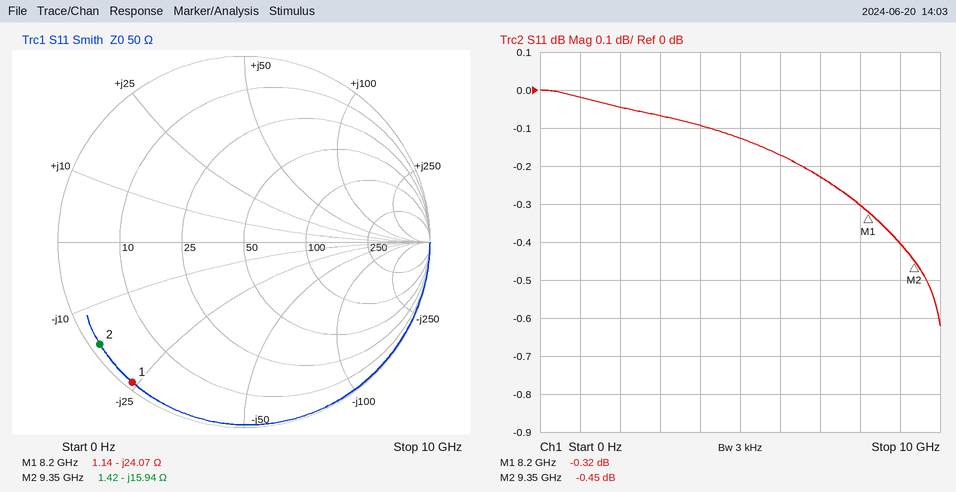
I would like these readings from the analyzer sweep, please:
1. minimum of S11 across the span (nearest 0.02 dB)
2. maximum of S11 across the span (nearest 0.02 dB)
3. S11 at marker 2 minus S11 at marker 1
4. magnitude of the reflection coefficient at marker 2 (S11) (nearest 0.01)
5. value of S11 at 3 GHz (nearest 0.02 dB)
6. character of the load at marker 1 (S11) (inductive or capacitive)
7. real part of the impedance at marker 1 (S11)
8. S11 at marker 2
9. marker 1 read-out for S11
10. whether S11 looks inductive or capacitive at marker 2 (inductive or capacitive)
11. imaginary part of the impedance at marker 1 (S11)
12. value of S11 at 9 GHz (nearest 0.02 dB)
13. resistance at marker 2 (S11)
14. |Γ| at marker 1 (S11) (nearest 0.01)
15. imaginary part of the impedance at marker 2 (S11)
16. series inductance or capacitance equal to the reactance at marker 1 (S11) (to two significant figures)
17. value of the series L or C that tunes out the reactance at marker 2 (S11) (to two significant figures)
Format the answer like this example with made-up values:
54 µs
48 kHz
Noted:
-0.62 dB
0.00 dB
-0.13 dB
0.95
-0.06 dB
capacitive
1.14 Ω
-0.45 dB
-0.32 dB
capacitive
-24.07 Ω
-0.40 dB
1.42 Ω
0.96
-15.94 Ω
810 fF
270 pH
